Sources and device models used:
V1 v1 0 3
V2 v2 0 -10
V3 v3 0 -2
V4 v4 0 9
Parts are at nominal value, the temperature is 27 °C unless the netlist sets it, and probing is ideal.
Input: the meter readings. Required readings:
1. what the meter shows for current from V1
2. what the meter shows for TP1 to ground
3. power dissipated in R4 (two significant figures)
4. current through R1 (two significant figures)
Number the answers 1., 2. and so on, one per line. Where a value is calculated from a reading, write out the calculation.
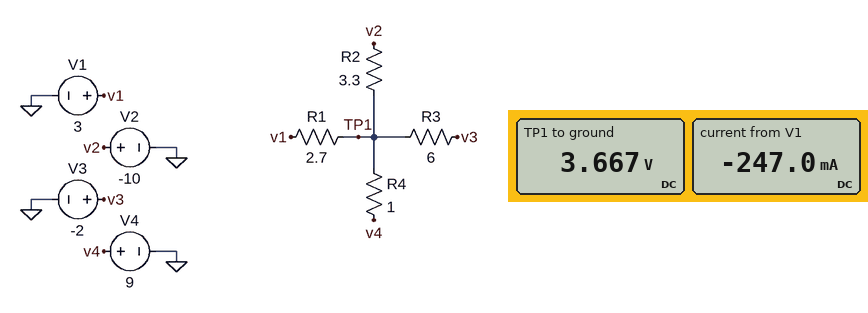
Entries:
1. -247.0 mA
2. 3.667 V
3. (9 V - 3.667 V)^2 / 1 Ω = 28 W
4. (3.667 V - 3 V) / 2.7 Ω = 250 mA
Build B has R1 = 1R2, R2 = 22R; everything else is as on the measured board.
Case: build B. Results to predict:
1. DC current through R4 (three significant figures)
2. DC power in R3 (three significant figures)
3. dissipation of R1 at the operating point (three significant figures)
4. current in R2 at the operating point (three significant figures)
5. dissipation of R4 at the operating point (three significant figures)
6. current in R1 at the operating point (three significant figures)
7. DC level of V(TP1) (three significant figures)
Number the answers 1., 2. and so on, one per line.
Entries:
1. 3.76 A
2. 8.73 W
3. 4.17 W
4. 693 mA
5. 14.2 W
6. 1.86 A
7. 5.24 V
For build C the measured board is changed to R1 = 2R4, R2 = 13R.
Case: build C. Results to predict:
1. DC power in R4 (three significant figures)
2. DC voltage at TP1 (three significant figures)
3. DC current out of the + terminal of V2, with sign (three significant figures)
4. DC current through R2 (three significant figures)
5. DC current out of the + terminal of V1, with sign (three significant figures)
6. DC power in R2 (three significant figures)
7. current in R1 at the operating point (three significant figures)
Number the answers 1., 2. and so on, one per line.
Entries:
1. 12.2 W
2. 5.51 V
3. -1.19 A
4. 1.19 A
5. -1.05 A
6. 18.5 W
7. 1.05 A
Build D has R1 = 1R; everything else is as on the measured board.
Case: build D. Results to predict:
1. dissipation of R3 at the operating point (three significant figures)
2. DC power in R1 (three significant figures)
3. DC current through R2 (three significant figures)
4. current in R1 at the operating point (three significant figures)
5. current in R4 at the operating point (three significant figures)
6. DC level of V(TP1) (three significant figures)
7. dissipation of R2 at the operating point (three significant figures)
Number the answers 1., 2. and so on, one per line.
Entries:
1. 5.04 W
2. 247 mW
3. 4.09 A
4. 497 mA
5. 5.50 A
6. 3.50 V
7. 55.2 W
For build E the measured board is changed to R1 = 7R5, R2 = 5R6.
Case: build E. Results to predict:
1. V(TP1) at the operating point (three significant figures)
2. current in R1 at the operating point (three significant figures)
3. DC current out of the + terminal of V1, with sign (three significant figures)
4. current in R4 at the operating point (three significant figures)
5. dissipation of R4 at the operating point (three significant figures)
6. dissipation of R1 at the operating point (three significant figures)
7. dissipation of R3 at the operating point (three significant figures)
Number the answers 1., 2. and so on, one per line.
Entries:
1. 4.92 V
2. 257 mA
3. -257 mA
4. 4.08 A
5. 16.6 W
6. 494 mW
7. 7.99 W
